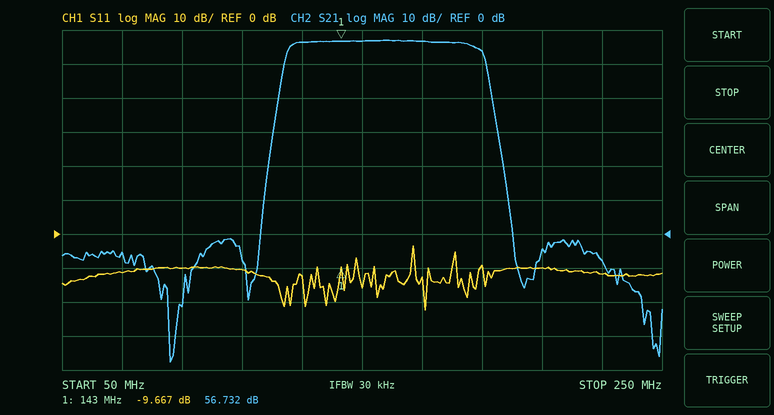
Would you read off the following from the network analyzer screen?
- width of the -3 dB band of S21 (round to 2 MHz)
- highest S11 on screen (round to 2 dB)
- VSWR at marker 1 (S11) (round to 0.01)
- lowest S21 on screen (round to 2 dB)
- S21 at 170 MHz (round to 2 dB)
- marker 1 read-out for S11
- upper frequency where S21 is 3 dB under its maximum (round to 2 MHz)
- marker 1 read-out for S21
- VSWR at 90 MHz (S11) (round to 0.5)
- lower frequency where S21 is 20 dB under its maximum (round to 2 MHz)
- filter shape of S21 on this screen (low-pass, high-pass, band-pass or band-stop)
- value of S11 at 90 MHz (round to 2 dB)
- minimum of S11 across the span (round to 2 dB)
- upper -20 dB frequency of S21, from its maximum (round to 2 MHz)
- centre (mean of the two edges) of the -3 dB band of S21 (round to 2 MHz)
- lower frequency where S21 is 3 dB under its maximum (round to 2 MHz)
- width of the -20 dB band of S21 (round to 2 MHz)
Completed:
64 MHz
-4 dB
1.98
-38 dB
56 dB
-9.667 dB
190 MHz
56.732 dB
2.0
122 MHz
band-pass
-10 dB
-22 dB
194 MHz
158 MHz
126 MHz
72 MHz
